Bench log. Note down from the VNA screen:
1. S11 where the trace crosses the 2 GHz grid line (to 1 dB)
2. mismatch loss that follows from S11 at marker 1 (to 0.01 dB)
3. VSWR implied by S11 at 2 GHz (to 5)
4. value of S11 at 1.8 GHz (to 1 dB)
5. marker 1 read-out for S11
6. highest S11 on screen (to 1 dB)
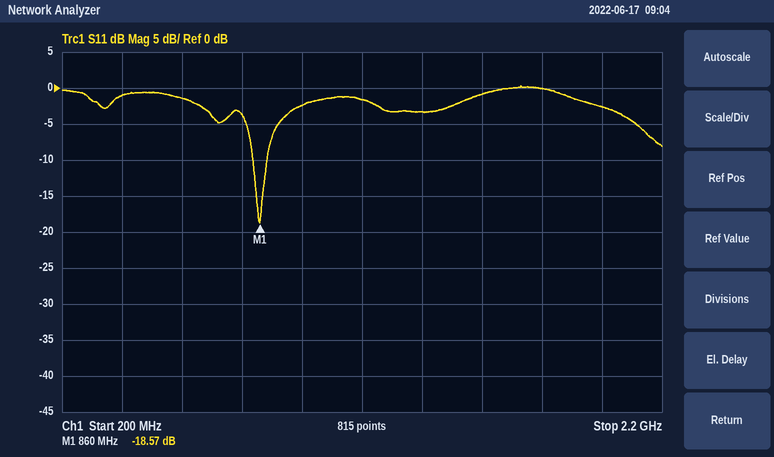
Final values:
-3 dB
0.06 dB
5
0 dB
-18.57 dB
0 dB
